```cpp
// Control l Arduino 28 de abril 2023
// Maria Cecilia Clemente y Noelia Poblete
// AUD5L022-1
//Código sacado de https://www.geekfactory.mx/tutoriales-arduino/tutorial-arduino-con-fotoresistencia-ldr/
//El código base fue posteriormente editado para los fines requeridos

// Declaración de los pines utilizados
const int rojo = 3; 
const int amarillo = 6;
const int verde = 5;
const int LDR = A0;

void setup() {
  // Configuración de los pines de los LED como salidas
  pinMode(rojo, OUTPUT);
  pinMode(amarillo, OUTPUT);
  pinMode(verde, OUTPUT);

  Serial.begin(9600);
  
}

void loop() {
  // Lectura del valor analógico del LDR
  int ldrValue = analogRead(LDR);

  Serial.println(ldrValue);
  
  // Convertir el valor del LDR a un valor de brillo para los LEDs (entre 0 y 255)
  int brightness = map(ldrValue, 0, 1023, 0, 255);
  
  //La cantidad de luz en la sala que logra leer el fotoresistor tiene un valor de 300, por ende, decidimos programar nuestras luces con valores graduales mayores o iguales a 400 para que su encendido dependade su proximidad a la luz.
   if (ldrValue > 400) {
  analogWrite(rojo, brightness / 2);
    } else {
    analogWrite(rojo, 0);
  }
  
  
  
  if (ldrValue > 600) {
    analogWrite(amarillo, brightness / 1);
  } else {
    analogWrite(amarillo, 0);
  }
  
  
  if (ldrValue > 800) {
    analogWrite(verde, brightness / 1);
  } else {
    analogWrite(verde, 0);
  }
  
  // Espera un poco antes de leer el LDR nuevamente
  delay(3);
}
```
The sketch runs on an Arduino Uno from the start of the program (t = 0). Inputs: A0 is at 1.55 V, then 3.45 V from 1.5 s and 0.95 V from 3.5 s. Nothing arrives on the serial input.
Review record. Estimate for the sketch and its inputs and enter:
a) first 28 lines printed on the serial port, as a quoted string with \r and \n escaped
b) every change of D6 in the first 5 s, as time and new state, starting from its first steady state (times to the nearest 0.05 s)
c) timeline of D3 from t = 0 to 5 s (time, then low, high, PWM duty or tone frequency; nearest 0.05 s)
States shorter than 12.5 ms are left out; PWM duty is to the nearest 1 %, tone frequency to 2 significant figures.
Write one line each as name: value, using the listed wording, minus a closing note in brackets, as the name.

first 28 lines printed on the serial port, as a quoted string with \r and \n escaped: "317\r\n317\r\n317\r\n317\r\n317\r\n317\r\n317\r\n317\r\n317\r\n317\r\n317\r\n317\r\n317\r\n317\r\n317\r\n317\r\n317\r\n317\r\n317\r\n317\r\n317\r\n317\r\n317\r\n317\r\n317\r\n317\r\n317\r\n317\r\n"
every change of D6 in the first 5 s, as time and new state, starting from its first steady state: 0 s low; 1.5 s PWM 69 %; 3.5 s low
timeline of D3 from t = 0 to 5 s: 0 s low; 1.5 s PWM 34 %; 3.5 s low
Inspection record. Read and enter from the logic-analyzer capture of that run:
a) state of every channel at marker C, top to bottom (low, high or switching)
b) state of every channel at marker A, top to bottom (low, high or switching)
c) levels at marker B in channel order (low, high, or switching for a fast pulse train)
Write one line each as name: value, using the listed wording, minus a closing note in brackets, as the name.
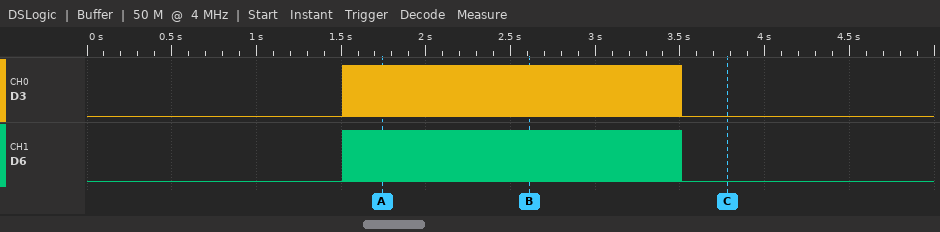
state of every channel at marker C, top to bottom: D3 low, D6 low
state of every channel at marker A, top to bottom: D3 switching, D6 switching
levels at marker B in channel order: D3 switching, D6 switching
